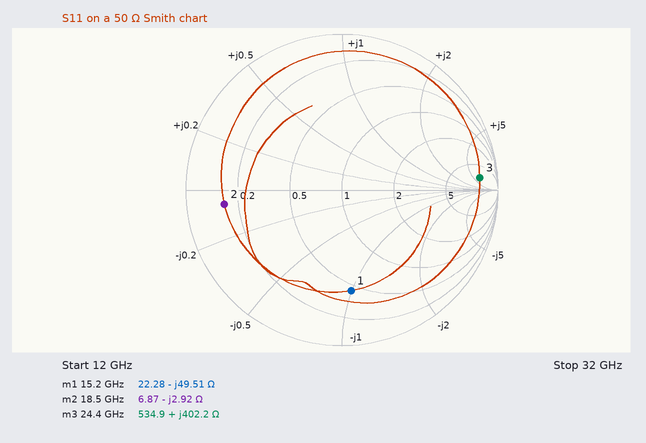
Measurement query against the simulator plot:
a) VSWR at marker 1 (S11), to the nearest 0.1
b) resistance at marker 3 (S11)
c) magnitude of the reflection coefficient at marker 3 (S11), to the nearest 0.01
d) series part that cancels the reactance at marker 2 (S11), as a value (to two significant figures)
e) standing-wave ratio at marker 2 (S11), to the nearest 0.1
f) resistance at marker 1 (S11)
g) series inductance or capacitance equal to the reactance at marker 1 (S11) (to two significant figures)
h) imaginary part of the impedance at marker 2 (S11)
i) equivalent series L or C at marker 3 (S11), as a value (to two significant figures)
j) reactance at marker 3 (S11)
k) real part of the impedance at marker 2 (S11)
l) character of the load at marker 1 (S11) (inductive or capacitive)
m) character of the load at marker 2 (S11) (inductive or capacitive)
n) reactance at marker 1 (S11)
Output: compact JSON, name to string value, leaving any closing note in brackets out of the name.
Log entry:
{"VSWR at marker 1 (S11), to the nearest 0.1": "4.7", "resistance at marker 3": "534.9 Ω", "magnitude of the reflection coefficient at marker 3 (S11), to the nearest 0.01": "0.89", "series part that cancels the reactance at marker 2 (S11), as a value": "25 pH", "standing-wave ratio at marker 2 (S11), to the nearest 0.1": "7.3", "resistance at marker 1": "22.28 Ω", "series inductance or capacitance equal to the reactance at marker 1 (S11)": "210 fF", "imaginary part of the impedance at marker 2": "-2.92 Ω", "equivalent series L or C at marker 3 (S11), as a value": "2.6 nH", "reactance at marker 3": "+402.2 Ω", "real part of the impedance at marker 2": "6.87 Ω", "character of the load at marker 1 (S11)": "capacitive", "character of the load at marker 2 (S11)": "capacitive", "reactance at marker 1": "-49.51 Ω"}
